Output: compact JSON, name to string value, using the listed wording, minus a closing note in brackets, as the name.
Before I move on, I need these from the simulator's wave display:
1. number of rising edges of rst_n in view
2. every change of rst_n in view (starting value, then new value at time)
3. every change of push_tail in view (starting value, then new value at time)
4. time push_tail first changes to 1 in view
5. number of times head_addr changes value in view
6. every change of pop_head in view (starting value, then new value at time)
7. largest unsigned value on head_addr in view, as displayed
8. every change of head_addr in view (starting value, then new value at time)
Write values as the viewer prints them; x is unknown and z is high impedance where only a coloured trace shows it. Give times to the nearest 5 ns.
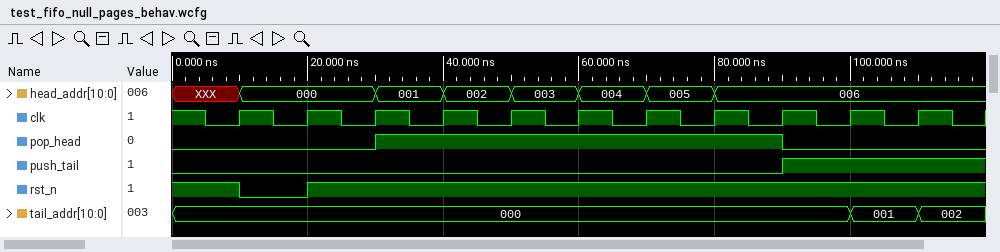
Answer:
{"number of rising edges of rst_n in view": "1", "every change of rst_n in view": "1, 0 at 10 ns, 1 at 20 ns", "every change of push_tail in view": "0, 1 at 90 ns", "time push_tail first changes to 1 in view": "90 ns", "number of times head_addr changes value in view": "7", "every change of pop_head in view": "0, 1 at 30 ns, 0 at 90 ns", "largest unsigned value on head_addr in view, as displayed": "006", "every change of head_addr in view": "XXX, 000 at 10 ns, 001 at 30 ns, 002 at 40 ns, 003 at 50 ns, 004 at 60 ns, 005 at 70 ns, 006 at 80 ns"}
